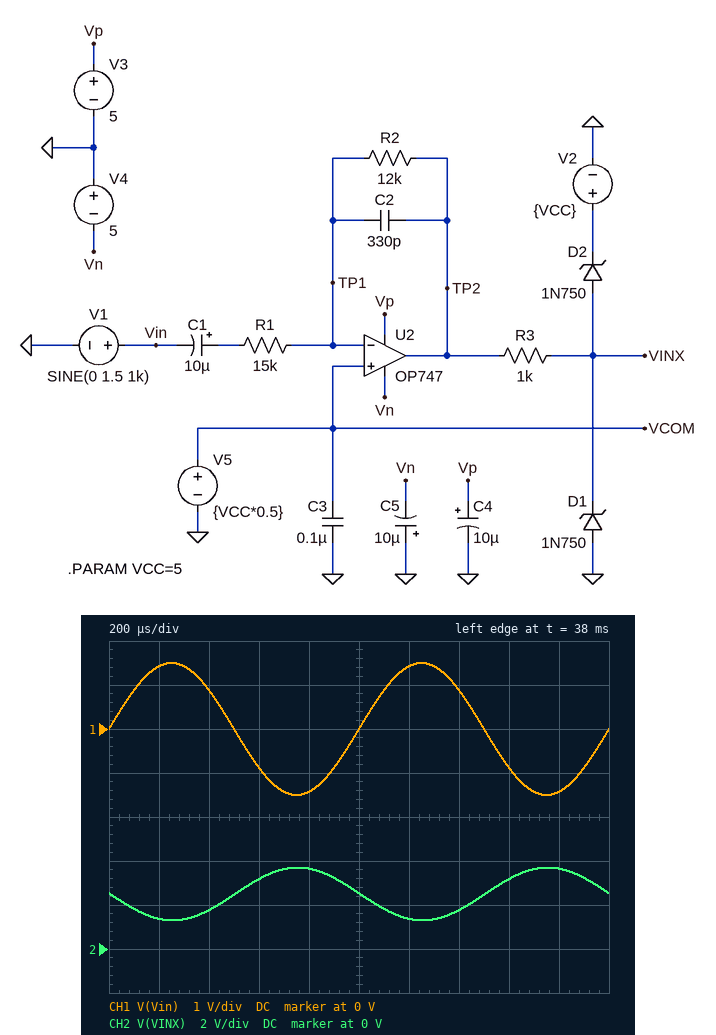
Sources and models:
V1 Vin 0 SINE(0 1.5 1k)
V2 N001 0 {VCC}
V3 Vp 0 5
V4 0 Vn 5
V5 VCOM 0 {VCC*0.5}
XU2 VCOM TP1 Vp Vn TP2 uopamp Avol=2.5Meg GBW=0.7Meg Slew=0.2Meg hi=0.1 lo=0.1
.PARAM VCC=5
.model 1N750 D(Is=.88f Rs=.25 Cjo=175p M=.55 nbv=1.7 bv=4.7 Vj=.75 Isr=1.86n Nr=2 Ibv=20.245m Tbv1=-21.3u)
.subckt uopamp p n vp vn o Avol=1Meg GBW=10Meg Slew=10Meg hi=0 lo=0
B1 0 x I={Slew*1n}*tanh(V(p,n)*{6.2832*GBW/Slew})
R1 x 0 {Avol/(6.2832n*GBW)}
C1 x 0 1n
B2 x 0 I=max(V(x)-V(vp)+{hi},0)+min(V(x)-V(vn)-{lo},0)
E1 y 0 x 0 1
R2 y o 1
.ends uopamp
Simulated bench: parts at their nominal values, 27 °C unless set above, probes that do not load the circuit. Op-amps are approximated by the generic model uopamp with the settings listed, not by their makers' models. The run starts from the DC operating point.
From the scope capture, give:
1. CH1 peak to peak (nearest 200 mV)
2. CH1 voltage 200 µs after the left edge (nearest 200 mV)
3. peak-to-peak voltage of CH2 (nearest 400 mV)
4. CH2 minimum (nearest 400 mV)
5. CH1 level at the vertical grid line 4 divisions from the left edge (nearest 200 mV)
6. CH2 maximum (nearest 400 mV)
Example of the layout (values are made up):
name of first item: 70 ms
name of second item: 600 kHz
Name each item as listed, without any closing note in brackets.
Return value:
CH1 peak to peak: 3.0 V
CH1 voltage 200 µs after the left edge: 1.4 V
peak-to-peak voltage of CH2: 2.4 V
CH2 minimum: 1.2 V
CH1 level at the vertical grid line 4 divisions from the left edge: -1.4 V
CH2 maximum: 3.6 V
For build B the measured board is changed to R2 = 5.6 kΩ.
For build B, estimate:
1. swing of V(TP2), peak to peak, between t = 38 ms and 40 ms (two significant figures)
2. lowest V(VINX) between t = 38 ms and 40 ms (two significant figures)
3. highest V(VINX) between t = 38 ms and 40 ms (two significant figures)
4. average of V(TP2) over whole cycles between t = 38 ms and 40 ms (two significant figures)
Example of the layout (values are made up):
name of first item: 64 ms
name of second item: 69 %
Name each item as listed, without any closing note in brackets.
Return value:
swing of V(TP2), peak to peak, between t = 38 ms and 40 ms: 1.1 V
lowest V(VINX) between t = 38 ms and 40 ms: 1.9 V
highest V(VINX) between t = 38 ms and 40 ms: 3.1 V
average of V(TP2) over whole cycles between t = 38 ms and 40 ms: 2.5 V
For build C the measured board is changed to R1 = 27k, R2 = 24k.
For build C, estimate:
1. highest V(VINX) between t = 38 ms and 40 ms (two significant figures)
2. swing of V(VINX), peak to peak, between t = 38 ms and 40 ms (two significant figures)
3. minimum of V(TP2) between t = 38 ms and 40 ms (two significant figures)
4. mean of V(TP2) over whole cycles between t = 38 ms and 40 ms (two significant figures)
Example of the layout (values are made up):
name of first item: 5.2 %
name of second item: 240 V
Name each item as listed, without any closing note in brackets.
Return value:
highest V(VINX) between t = 38 ms and 40 ms: 3.8 V
swing of V(VINX), peak to peak, between t = 38 ms and 40 ms: 2.7 V
minimum of V(TP2) between t = 38 ms and 40 ms: 1.2 V
mean of V(TP2) over whole cycles between t = 38 ms and 40 ms: 2.5 V
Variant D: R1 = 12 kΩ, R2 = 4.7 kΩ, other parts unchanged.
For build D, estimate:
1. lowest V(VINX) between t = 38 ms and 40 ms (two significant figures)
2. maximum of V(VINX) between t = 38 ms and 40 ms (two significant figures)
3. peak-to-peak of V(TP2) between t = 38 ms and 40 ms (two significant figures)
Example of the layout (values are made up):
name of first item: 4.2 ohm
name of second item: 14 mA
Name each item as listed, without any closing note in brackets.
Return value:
lowest V(VINX) between t = 38 ms and 40 ms: 1.9 V
maximum of V(VINX) between t = 38 ms and 40 ms: 3.1 V
peak-to-peak of V(TP2) between t = 38 ms and 40 ms: 1.2 V
